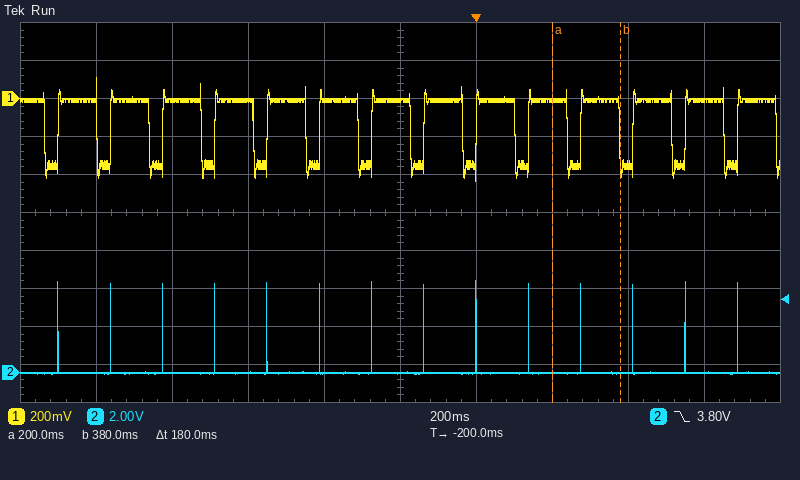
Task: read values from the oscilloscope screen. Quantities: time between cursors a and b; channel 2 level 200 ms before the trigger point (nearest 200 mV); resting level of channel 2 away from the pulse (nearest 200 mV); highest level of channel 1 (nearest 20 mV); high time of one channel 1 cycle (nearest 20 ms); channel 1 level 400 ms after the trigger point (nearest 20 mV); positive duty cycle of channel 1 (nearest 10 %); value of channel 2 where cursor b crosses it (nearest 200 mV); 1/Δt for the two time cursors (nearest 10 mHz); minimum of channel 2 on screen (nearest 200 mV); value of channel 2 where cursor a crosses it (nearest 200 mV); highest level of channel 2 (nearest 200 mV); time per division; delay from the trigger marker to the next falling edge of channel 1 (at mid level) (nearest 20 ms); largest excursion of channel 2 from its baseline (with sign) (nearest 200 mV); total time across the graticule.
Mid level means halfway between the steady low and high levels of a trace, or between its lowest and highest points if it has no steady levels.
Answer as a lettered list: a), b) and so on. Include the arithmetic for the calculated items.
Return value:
a) 180 ms
b) 0.0 V
c) 0.0 V
d) 120 mV
e) 100 ms
f) -340 mV
g) 70 %
h) 0.0 V
i) 1 / 180 ms ≈ 5.56 Hz
j) 0.0 V
k) 0.0 V
l) 4.8 V
m) 200 ms
n) 100 ms
o) 4.8 V − (0.0 V) = +4.8 V
p) 2 s
